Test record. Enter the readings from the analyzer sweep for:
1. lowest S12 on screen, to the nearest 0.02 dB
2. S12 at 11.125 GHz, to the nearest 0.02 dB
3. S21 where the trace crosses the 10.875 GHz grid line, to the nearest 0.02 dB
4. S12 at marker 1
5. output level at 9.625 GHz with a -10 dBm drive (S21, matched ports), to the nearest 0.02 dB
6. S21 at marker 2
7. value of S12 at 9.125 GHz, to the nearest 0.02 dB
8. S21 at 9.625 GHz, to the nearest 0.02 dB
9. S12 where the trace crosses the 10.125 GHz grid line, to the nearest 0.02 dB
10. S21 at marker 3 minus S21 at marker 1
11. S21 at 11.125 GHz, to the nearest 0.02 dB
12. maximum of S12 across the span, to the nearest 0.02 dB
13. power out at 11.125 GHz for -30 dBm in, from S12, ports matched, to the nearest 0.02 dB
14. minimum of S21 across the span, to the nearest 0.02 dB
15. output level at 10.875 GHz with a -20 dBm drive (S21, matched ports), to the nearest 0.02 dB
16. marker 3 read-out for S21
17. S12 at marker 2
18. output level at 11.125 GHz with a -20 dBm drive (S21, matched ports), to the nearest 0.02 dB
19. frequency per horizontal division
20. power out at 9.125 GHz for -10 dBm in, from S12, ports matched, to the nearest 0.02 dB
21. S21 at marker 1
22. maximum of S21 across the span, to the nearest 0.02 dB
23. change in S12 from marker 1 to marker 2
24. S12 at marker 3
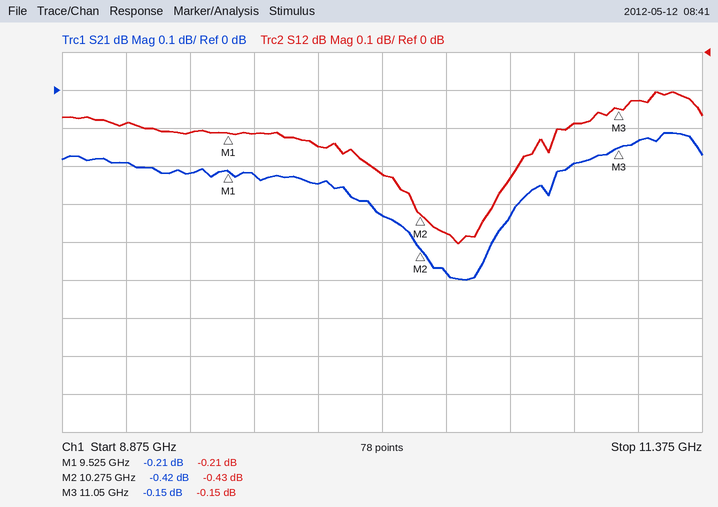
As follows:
-0.50 dB
-0.12 dB
-0.20 dB
-0.21 dB
-10.22 dBm
-0.42 dB
-0.18 dB
-0.22 dB
-0.32 dB
0.06 dB
-0.14 dB
-0.10 dB
-30.12 dBm
-0.50 dB
-20.20 dBm
-0.15 dB
-0.43 dB
-20.14 dBm
250 MHz
-10.18 dBm
-0.21 dB
-0.12 dB
-0.22 dB
-0.15 dB
